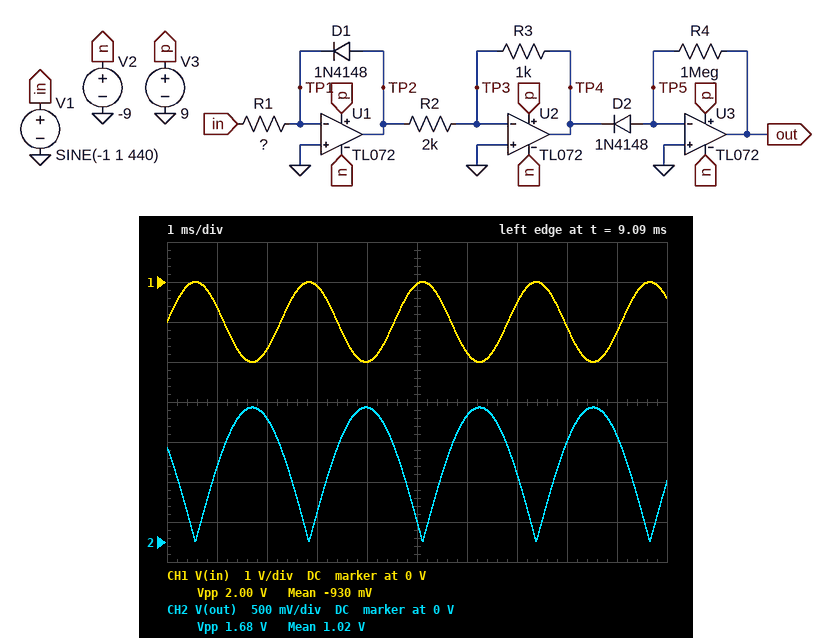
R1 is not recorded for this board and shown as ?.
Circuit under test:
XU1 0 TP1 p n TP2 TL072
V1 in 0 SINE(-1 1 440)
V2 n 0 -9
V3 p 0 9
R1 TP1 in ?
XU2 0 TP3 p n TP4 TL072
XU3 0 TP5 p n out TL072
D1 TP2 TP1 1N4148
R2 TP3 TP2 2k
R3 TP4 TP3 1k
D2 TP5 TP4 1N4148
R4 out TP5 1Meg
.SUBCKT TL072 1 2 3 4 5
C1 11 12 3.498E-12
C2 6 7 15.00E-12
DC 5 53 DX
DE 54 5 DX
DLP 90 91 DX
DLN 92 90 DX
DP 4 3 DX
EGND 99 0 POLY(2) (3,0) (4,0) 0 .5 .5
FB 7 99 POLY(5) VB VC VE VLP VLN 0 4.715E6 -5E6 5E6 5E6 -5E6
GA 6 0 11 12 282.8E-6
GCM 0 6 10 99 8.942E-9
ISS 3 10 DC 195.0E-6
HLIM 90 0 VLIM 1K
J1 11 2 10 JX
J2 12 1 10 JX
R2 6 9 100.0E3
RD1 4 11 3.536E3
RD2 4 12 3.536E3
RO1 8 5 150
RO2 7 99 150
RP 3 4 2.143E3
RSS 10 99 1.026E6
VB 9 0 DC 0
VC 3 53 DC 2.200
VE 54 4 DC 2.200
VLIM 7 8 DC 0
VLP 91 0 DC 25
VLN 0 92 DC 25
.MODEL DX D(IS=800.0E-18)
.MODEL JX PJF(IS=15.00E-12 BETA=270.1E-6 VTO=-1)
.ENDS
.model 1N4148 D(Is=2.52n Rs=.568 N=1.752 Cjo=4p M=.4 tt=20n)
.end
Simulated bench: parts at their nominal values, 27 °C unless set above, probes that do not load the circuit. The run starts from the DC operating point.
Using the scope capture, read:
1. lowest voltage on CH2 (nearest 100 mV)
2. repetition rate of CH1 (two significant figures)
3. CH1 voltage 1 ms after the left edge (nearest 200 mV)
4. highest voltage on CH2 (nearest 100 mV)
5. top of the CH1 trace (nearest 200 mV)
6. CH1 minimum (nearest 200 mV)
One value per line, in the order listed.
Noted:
0 V
440 Hz
-600 mV
1.7 V
0 V
-2.0 V
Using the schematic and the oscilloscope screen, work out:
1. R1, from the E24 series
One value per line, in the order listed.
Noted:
1.8 kΩ
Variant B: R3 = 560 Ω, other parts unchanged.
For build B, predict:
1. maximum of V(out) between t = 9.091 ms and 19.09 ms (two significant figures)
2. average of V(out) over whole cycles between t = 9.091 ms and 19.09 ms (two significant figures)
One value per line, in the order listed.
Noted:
94 mV
69 mV
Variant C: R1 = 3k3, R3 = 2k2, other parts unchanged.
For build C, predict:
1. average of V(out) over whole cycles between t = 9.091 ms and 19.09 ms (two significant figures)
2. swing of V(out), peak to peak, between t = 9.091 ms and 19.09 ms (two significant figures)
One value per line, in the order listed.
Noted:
7.2 V
7.4 V
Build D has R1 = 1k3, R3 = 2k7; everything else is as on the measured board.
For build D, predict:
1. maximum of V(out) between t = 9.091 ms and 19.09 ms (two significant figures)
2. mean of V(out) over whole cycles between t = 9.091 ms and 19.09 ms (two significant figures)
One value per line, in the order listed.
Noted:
7.5 V
7.4 V
